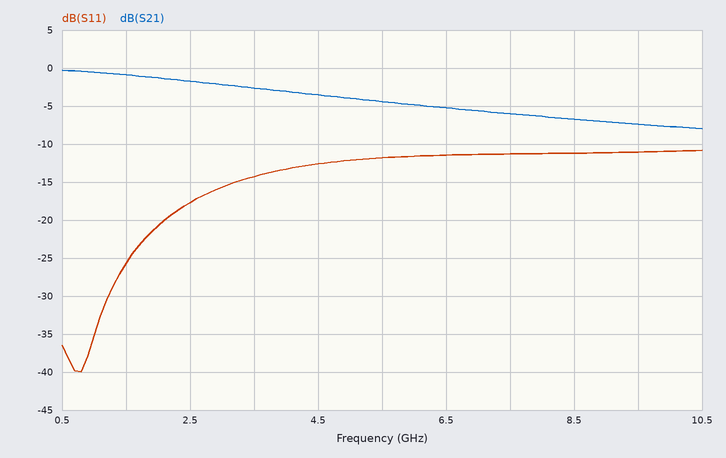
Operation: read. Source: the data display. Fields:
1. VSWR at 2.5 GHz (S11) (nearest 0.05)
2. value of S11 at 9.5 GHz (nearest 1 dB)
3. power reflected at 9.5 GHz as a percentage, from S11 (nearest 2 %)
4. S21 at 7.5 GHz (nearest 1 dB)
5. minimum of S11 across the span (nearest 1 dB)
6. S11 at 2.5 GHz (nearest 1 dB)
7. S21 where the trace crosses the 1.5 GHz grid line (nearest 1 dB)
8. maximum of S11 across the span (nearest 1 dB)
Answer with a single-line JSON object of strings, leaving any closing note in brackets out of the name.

{"VSWR at 2.5 GHz (S11)": "1.30", "value of S11 at 9.5 GHz": "-11 dB", "power reflected at 9.5 GHz as a percentage, from S11": "8 %", "S21 at 7.5 GHz": "-6 dB", "minimum of S11 across the span": "-40 dB", "S11 at 2.5 GHz": "-18 dB", "S21 where the trace crosses the 1.5 GHz grid line": "-1 dB", "maximum of S11 across the span": "-11 dB"}
